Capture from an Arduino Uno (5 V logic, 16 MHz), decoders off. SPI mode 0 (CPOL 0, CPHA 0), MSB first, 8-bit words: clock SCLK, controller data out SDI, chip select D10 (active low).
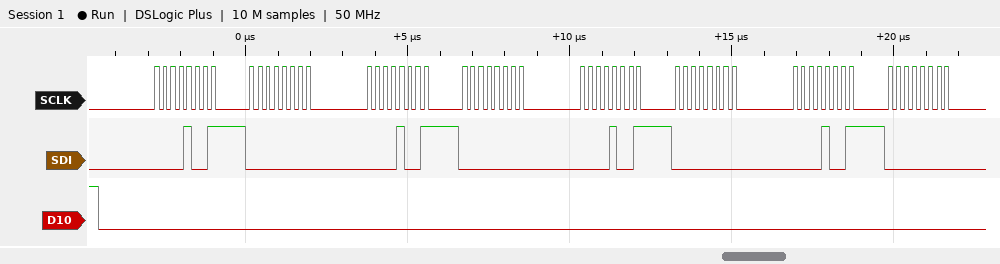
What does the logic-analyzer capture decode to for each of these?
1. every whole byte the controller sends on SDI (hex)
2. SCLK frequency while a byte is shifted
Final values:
09 00 09 00 09 00 09 00
4 MHz
